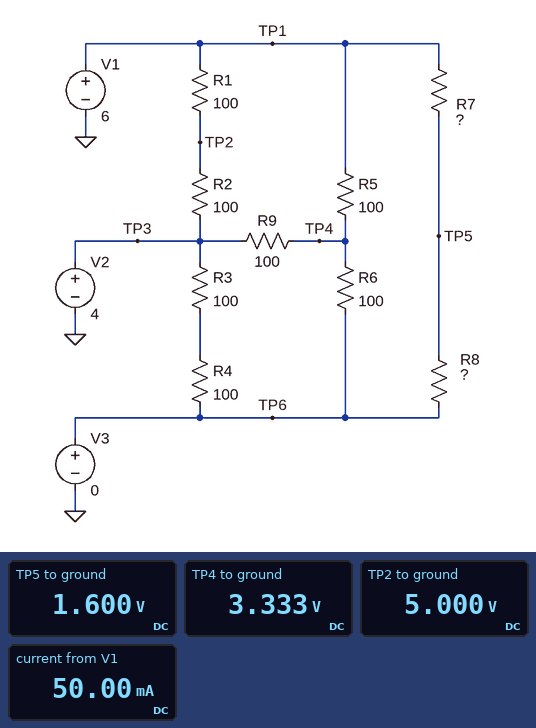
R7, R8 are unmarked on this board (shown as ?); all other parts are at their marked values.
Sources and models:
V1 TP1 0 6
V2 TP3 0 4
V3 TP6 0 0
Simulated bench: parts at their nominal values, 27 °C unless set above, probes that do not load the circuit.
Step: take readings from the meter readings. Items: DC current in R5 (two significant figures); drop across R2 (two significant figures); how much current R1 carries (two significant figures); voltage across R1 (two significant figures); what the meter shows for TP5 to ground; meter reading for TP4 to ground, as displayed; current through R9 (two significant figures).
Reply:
27 mA
1.0 V
10 mA
1.0 V
1.600 V
3.333 V
6.7 mA
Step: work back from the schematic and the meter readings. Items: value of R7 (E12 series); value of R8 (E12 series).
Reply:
330 Ω
120 Ω
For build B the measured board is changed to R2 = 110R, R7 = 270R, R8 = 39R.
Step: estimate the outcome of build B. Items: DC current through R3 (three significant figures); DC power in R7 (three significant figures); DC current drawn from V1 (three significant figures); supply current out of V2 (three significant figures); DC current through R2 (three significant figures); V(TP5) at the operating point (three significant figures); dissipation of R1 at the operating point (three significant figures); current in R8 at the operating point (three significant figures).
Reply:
20.0 mA
102 mW
55.6 mA
17.1 mA
9.52 mA
757 mV
9.07 mW
19.4 mA
